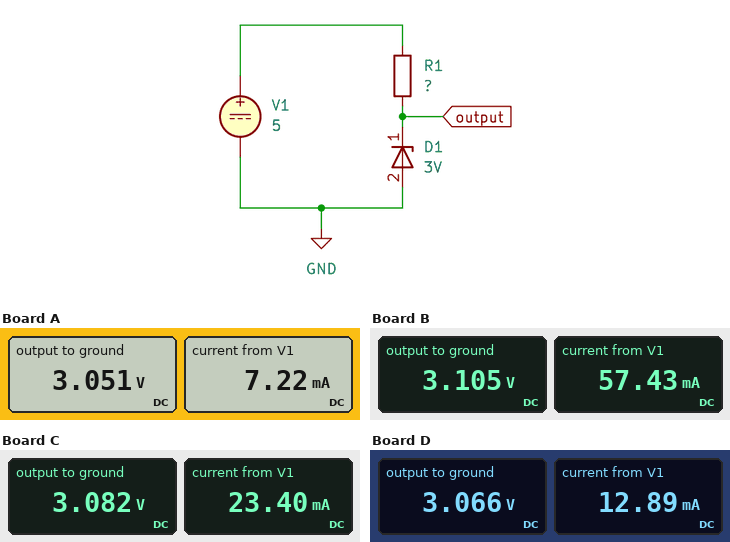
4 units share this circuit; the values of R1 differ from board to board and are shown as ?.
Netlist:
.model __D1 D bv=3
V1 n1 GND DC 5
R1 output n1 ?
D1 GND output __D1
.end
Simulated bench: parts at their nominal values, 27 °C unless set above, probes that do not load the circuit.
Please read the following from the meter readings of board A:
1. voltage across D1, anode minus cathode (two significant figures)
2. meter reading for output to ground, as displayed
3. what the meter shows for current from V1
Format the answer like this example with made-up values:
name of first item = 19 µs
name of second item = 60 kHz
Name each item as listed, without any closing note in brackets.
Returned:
voltage across D1, anode minus cathode = -3.1 V
meter reading for output to ground, as displayed = 3.051 V
what the meter shows for current from V1 = 7.22 mA
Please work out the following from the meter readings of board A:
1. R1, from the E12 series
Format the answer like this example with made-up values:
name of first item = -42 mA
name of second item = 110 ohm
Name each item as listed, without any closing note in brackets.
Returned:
R1, from the E12 series = 270 Ω
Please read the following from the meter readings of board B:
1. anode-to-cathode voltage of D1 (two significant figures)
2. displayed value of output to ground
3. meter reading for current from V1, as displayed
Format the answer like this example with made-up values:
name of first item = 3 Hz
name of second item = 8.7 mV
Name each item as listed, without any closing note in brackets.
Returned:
anode-to-cathode voltage of D1 = -3.1 V
displayed value of output to ground = 3.105 V
meter reading for current from V1, as displayed = 57.43 mA
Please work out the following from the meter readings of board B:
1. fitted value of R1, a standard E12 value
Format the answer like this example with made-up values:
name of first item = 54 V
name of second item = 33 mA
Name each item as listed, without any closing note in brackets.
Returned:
fitted value of R1, a standard E12 value = 33 Ω
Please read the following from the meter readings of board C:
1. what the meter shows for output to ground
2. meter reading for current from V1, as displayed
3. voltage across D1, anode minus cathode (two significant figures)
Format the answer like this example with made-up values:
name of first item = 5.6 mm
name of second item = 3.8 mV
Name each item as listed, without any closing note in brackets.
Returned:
what the meter shows for output to ground = 3.082 V
meter reading for current from V1, as displayed = 23.40 mA
voltage across D1, anode minus cathode = -3.1 V
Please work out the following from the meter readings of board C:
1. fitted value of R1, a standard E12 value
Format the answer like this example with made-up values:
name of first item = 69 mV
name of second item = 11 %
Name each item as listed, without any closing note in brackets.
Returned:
fitted value of R1, a standard E12 value = 82 Ω
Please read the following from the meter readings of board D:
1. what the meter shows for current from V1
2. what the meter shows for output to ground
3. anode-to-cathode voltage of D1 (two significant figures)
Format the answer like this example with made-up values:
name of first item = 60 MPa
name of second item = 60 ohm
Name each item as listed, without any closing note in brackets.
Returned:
what the meter shows for current from V1 = 12.89 mA
what the meter shows for output to ground = 3.066 V
anode-to-cathode voltage of D1 = -3.1 V
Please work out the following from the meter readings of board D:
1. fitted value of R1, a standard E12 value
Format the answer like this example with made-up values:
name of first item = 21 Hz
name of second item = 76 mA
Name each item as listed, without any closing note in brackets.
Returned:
fitted value of R1, a standard E12 value = 150 Ω
